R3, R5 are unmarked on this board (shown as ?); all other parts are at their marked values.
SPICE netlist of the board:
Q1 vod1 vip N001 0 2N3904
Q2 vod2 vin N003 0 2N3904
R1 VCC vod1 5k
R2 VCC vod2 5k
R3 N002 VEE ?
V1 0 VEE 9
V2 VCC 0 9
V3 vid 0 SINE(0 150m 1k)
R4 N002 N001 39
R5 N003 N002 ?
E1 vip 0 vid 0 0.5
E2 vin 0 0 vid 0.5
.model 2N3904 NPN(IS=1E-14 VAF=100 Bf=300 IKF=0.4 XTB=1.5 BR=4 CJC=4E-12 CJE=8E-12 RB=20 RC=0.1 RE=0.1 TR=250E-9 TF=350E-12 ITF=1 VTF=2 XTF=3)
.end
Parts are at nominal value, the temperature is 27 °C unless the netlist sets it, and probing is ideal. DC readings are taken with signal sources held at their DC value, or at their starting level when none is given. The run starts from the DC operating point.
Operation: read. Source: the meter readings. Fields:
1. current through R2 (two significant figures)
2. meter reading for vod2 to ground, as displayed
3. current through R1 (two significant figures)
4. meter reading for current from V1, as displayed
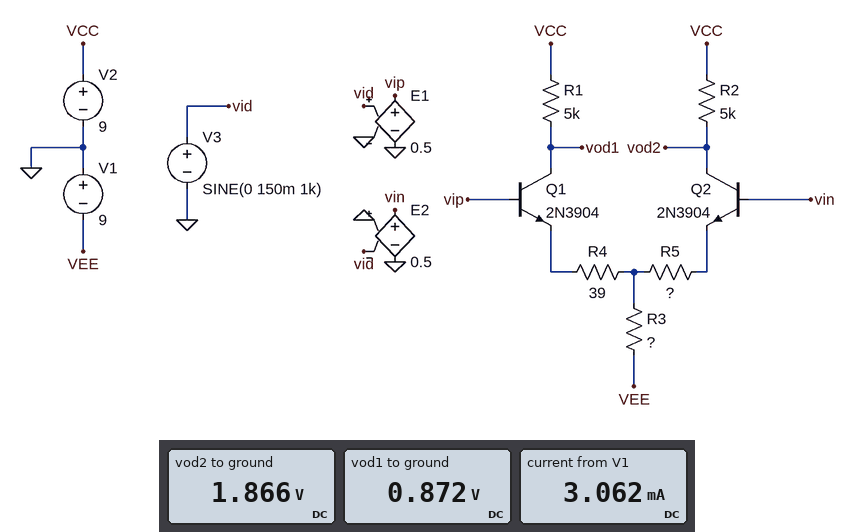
1.4 mA
1.866 V
1.6 mA
3.062 mA
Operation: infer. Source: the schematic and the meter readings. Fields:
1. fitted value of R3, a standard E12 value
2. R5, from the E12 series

2.7 kΩ
47 Ω
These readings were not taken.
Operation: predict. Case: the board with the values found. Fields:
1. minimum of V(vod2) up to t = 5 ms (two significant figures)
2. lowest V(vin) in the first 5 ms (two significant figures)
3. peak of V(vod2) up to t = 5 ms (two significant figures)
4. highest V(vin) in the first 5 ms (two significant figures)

-610 mV
-75 mV
6.5 V
75 mV
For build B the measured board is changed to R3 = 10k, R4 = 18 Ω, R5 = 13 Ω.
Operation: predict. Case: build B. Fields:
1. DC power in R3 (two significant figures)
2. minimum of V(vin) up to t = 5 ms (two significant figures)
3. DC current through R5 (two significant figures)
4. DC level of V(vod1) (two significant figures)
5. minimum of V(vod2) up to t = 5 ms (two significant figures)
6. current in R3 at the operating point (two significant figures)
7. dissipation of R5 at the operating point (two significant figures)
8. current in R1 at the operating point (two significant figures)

7.0 mW
-75 mV
430 µA
7.0 V
4.8 V
840 µA
2.4 µW
400 µA
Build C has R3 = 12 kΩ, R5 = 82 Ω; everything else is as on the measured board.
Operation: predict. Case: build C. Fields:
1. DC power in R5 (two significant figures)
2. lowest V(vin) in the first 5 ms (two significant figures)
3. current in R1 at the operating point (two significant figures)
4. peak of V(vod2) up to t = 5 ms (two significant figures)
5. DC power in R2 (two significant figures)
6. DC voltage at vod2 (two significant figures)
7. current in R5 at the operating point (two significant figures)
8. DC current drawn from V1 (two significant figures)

7.1 µW
-75 mV
400 µA
9.0 V
430 µW
7.5 V
290 µA
700 µA
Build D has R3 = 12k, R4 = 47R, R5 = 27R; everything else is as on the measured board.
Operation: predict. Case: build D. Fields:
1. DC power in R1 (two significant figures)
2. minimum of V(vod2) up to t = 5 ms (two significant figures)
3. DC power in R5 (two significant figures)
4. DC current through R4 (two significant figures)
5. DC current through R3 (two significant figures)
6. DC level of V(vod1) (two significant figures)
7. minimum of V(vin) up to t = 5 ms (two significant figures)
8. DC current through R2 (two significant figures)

500 µW
5.5 V
3.9 µW
320 µA
700 µA
7.4 V
-75 mV
380 µA
